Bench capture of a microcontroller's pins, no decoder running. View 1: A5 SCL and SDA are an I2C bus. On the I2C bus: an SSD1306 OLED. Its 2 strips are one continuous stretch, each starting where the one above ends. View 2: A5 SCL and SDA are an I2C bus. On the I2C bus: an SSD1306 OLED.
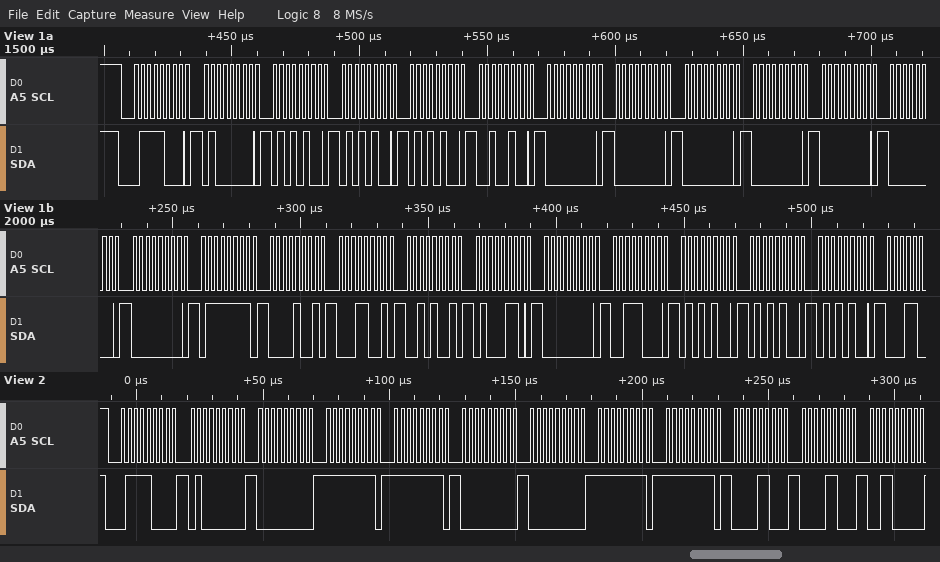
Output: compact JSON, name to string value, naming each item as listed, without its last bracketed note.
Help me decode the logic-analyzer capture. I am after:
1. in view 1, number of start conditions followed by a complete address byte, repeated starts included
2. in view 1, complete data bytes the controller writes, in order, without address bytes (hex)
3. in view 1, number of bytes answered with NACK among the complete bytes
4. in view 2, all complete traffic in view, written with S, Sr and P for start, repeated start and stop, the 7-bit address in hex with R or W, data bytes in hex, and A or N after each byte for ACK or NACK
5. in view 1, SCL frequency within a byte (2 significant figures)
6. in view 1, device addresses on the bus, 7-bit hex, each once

{"in view 1, number of start conditions followed by a complete address byte, repeated starts included": "1", "in view 1, complete data bytes the controller writes, in order, without address bytes": "40 54 54 54 24 00 00 00 00 00 00 00 7F 09 19 29 46 00 38 54 54 54", "in view 1, number of bytes answered with NACK among the complete bytes": "0", "in view 2, all complete traffic in view, written with S, Sr and P for start, repeated start and stop, the 7-bit address in hex with R or W, data bytes in hex, and A or N after each byte for ACK or NACK": "S 3CW A 40 A 00 A FF A FF A 00 A 00 A FF A FF A 0C A 0C A 30 A", "in view 1, SCL frequency within a byte": "400 kHz", "in view 1, device addresses on the bus, 7-bit hex, each once": "0x3C"}
